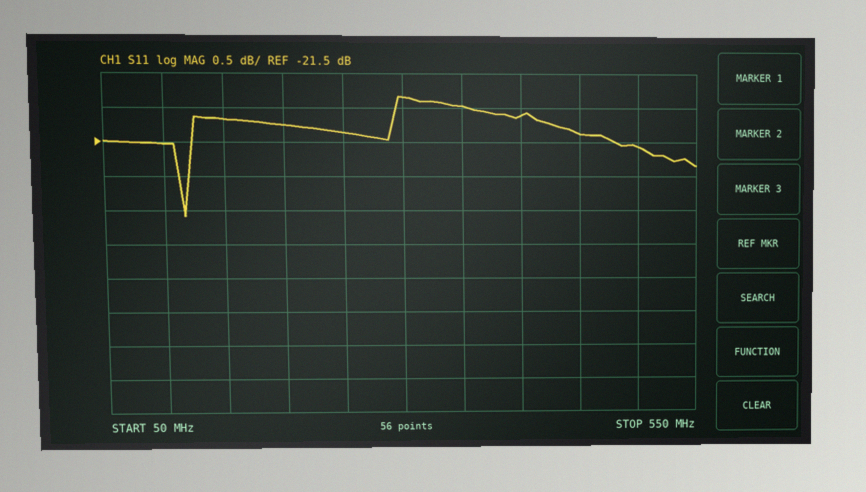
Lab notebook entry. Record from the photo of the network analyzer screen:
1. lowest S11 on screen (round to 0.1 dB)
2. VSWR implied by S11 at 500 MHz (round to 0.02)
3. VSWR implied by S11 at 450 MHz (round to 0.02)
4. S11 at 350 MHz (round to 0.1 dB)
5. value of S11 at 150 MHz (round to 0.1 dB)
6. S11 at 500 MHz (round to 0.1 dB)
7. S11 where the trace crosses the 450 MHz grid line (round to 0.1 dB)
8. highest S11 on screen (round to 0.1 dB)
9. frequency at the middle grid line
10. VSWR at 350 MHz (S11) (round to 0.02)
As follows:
-22.6 dB
1.18
1.18
-21.0 dB
-21.2 dB
-21.6 dB
-21.4 dB
-20.8 dB
300 MHz
1.20
